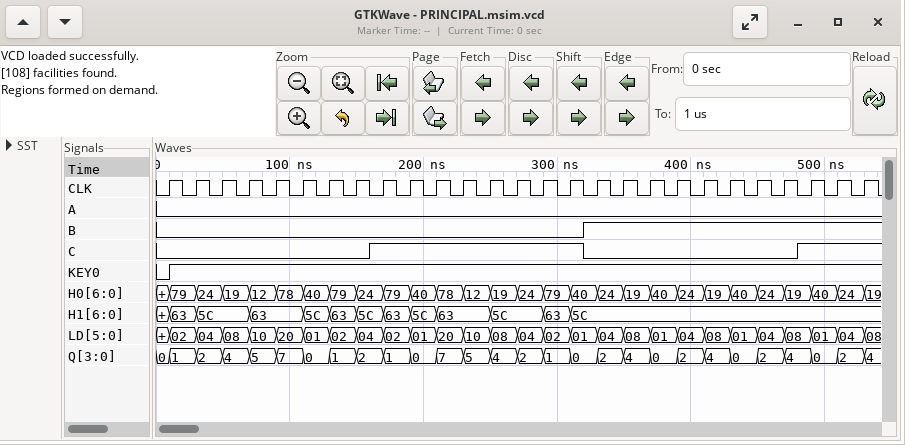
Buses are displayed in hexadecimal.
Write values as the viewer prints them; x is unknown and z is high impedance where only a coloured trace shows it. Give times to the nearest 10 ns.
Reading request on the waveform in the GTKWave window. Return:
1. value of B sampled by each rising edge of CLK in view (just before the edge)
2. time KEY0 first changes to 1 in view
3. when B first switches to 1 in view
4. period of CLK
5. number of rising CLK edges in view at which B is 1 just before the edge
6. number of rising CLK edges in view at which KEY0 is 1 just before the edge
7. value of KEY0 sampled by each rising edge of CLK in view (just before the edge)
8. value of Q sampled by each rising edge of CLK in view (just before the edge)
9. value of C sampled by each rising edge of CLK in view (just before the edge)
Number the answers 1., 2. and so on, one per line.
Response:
1. 0 0 0 0 0 0 0 0 0 0 0 0 0 0 0 0 1 1 1 1 1 1 1 1 1 1 1
2. 10 ns
3. 320 ns
4. 20 ns
5. 11
6. 26
7. 0 1 1 1 1 1 1 1 1 1 1 1 1 1 1 1 1 1 1 1 1 1 1 1 1 1 1
8. 0, 1, 2, 4, 5, 7, 0, 1, 2, 1, 0, 7, 5, 4, 2, 1, 0, 2, 4, 0, 2, 4, 0, 2, 4, 0, 2
9. 0 0 0 0 0 0 0 0 1 1 1 1 1 1 1 1 0 0 0 0 0 0 0 0 1 1 1
